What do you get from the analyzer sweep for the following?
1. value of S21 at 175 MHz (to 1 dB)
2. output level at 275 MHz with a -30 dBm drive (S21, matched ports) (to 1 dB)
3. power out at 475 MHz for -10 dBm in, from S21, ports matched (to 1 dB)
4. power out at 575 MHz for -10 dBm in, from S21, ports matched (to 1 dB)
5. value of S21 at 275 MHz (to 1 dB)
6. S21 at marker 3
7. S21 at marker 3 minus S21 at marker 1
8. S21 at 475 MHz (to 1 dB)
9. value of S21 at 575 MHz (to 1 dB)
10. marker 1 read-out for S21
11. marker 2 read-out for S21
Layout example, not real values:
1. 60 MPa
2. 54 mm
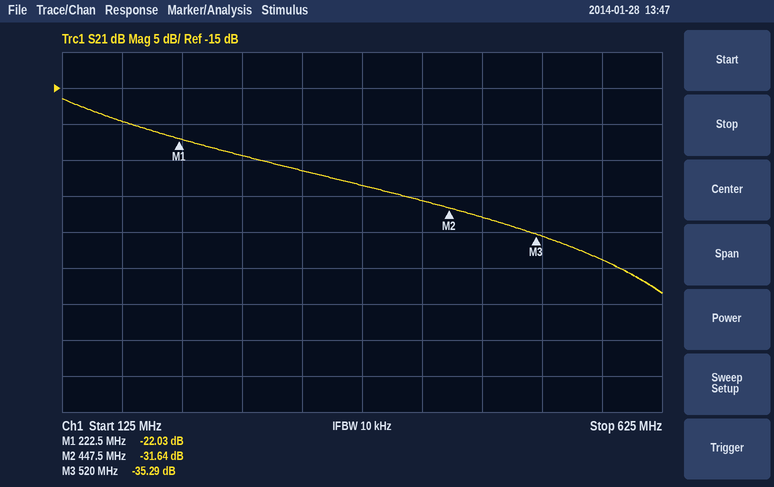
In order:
1. -20 dB
2. -54 dBm
3. -43 dBm
4. -49 dBm
5. -24 dB
6. -35.29 dB
7. -13.26 dB
8. -33 dB
9. -39 dB
10. -22.03 dB
11. -31.64 dB
